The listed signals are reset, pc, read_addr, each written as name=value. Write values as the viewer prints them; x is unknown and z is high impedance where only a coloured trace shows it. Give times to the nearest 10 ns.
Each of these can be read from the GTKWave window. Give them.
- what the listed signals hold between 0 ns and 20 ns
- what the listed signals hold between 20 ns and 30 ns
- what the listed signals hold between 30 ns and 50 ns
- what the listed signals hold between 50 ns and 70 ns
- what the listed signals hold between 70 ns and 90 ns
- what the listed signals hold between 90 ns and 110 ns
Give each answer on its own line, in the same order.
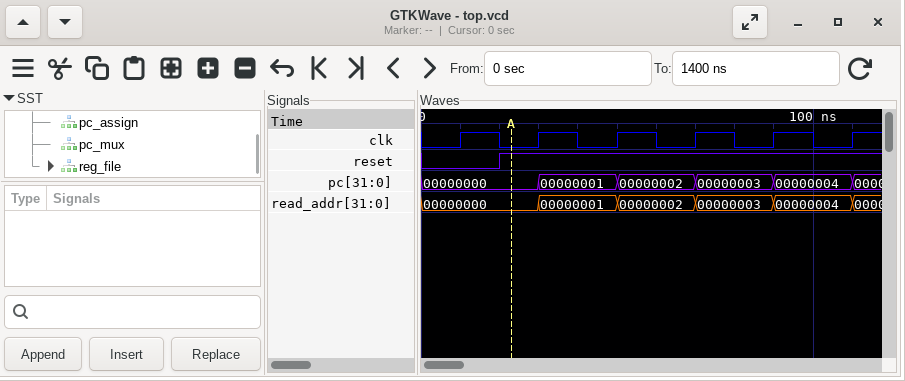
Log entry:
reset=0, pc=00000000, read_addr=00000000
reset=1, pc=00000000, read_addr=00000000
reset=1, pc=00000001, read_addr=00000001
reset=1, pc=00000002, read_addr=00000002
reset=1, pc=00000003, read_addr=00000003
reset=1, pc=00000004, read_addr=00000004
